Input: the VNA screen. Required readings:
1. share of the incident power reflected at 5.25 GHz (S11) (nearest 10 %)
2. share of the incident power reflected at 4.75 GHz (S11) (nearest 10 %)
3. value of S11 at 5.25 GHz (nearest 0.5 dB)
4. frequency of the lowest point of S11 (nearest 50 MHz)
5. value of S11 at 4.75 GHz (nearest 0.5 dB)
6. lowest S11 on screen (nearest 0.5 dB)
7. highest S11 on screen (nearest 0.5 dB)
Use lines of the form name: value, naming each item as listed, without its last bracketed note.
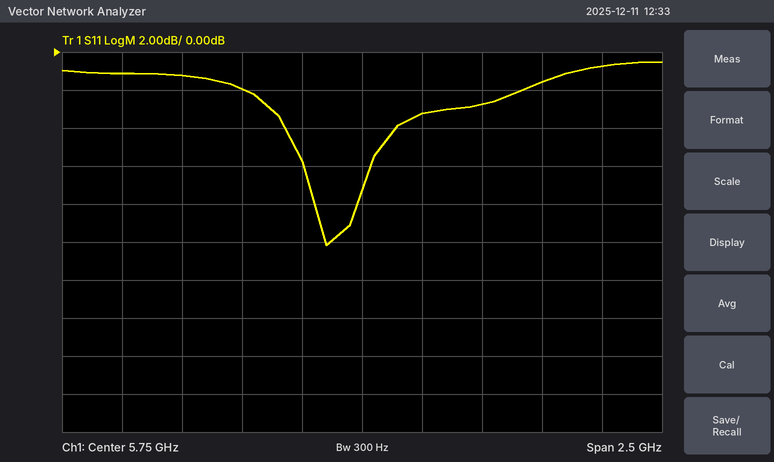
share of the incident power reflected at 5.25 GHz (S11): 60 %
share of the incident power reflected at 4.75 GHz (S11): 80 %
value of S11 at 5.25 GHz: -2.0 dB
frequency of the lowest point of S11: 5.60 GHz
value of S11 at 4.75 GHz: -1.0 dB
lowest S11 on screen: -10.0 dB
highest S11 on screen: -0.5 dB
